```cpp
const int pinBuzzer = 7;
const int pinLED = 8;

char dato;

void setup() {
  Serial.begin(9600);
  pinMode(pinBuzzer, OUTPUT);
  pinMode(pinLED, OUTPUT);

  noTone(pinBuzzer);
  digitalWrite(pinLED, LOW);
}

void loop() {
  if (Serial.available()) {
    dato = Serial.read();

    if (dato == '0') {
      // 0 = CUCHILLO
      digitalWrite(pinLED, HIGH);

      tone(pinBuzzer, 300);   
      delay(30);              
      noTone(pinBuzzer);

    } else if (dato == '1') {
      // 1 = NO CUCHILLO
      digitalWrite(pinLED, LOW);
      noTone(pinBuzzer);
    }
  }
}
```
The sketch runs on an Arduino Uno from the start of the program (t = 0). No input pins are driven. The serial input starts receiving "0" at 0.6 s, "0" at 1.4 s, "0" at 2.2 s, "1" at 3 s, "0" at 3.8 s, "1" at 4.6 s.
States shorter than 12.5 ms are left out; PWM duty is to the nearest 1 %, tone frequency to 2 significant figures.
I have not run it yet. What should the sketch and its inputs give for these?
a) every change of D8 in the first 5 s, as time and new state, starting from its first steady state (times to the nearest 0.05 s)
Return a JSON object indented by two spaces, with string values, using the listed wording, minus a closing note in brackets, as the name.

{
  "every change of D8 in the first 5 s, as time and new state, starting from its first steady state": "0 s low; 0.6 s high; 3 s low; 3.8 s high; 4.6 s low"
}
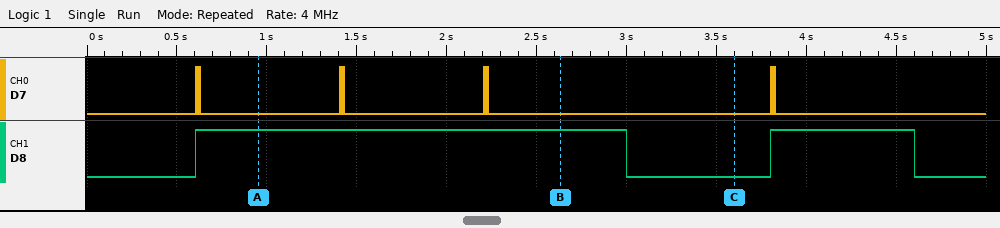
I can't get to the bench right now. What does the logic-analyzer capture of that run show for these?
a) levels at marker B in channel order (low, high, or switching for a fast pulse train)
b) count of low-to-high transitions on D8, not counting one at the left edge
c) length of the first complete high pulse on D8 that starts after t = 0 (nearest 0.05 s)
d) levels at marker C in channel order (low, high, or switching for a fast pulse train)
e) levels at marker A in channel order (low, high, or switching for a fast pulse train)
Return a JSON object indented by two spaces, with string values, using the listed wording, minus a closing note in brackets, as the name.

{
  "levels at marker B in channel order": "D7 low, D8 high",
  "count of low-to-high transitions on D8, not counting one at the left edge": "2",
  "length of the first complete high pulse on D8 that starts after t = 0": "2.40 s",
  "levels at marker C in channel order": "D7 low, D8 low",
  "levels at marker A in channel order": "D7 low, D8 high"
}
